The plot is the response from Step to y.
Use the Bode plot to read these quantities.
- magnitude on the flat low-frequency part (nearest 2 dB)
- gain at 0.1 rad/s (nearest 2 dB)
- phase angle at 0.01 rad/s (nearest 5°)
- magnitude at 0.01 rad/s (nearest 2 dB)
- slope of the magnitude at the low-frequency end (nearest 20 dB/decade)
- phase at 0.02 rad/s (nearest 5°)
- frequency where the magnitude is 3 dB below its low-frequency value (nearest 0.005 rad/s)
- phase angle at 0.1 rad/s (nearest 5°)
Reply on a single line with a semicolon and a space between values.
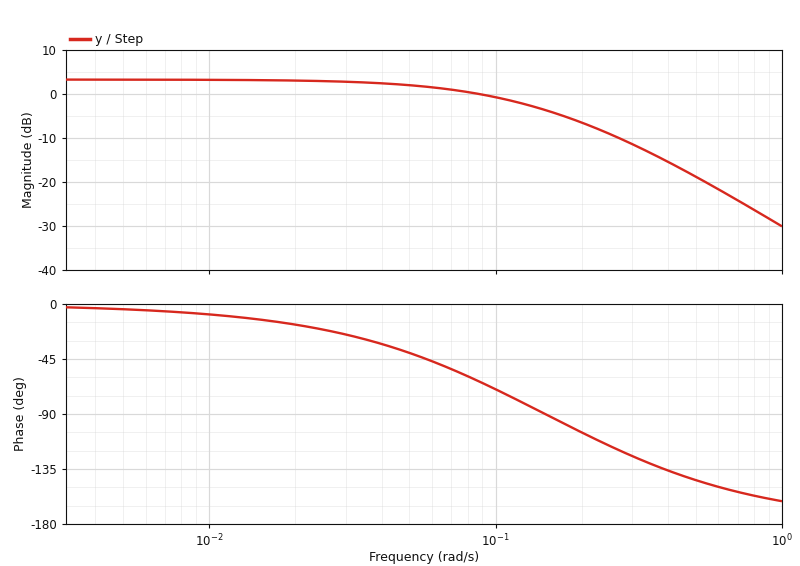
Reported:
4 dB; 0 dB; -10°; 4 dB; 0 dB/decade; -15°; 0.085 rad/s; -70°
